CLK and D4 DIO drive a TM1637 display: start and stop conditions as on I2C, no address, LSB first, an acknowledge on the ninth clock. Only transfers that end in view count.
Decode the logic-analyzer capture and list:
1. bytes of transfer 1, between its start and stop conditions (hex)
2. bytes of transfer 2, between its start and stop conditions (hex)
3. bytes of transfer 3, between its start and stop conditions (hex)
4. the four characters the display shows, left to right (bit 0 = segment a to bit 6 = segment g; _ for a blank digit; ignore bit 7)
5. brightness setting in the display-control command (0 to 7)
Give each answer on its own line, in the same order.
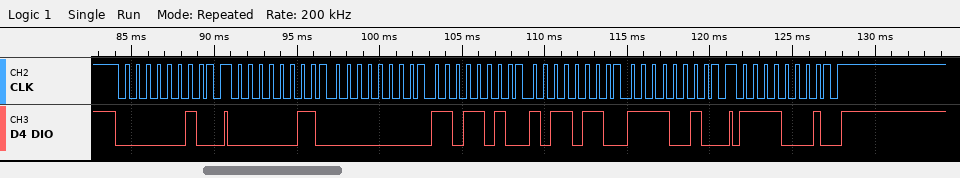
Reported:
40
C0 00 5B 6D 4F
8F
_253
7
